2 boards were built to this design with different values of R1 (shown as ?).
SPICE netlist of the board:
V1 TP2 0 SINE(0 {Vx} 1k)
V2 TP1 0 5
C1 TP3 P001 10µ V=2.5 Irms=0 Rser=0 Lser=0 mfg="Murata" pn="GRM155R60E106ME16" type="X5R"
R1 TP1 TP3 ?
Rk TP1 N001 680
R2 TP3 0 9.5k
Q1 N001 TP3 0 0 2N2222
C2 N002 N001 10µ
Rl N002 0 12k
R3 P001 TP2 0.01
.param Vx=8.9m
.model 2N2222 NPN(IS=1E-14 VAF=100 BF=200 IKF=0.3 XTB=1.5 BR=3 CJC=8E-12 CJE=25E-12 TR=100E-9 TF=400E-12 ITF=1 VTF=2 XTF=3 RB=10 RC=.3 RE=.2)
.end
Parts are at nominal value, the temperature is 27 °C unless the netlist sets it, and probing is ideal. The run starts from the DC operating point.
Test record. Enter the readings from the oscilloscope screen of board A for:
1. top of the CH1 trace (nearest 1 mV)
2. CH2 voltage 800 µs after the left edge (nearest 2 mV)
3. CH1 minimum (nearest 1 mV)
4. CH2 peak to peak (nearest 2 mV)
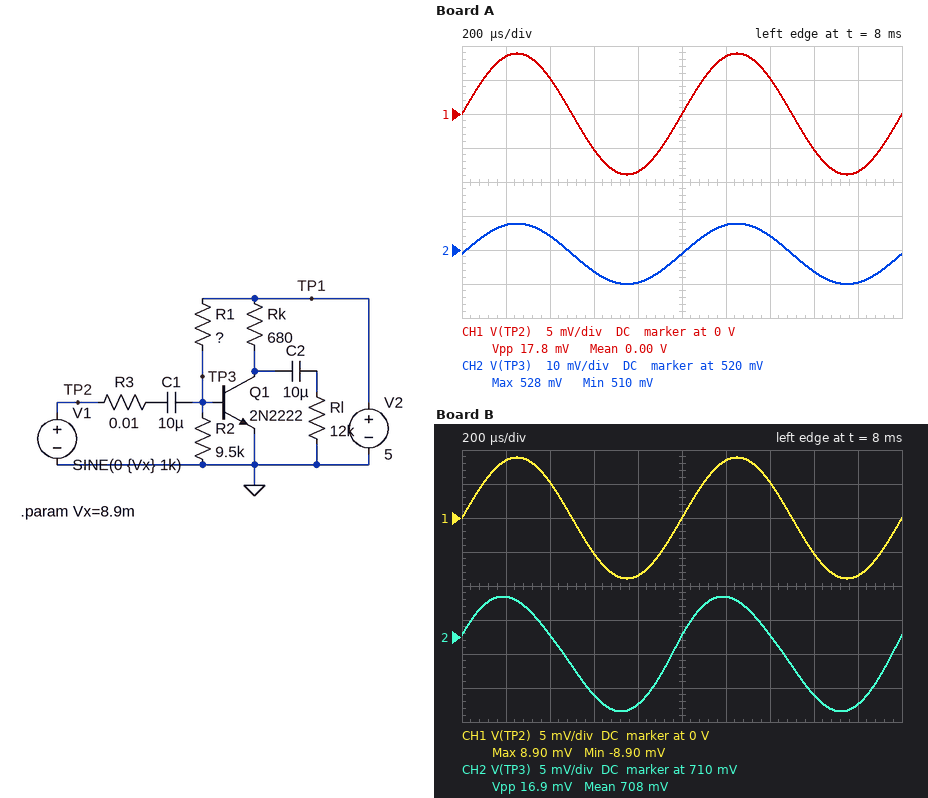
9 mV
510 mV
-9 mV
18 mV
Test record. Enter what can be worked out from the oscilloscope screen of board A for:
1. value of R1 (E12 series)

82 kΩ
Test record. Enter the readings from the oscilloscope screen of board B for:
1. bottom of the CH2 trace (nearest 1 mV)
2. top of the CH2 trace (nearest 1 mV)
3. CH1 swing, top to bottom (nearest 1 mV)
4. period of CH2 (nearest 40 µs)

699 mV
716 mV
18 mV
1.00 ms
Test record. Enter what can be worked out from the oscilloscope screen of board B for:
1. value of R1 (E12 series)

22 kΩ
